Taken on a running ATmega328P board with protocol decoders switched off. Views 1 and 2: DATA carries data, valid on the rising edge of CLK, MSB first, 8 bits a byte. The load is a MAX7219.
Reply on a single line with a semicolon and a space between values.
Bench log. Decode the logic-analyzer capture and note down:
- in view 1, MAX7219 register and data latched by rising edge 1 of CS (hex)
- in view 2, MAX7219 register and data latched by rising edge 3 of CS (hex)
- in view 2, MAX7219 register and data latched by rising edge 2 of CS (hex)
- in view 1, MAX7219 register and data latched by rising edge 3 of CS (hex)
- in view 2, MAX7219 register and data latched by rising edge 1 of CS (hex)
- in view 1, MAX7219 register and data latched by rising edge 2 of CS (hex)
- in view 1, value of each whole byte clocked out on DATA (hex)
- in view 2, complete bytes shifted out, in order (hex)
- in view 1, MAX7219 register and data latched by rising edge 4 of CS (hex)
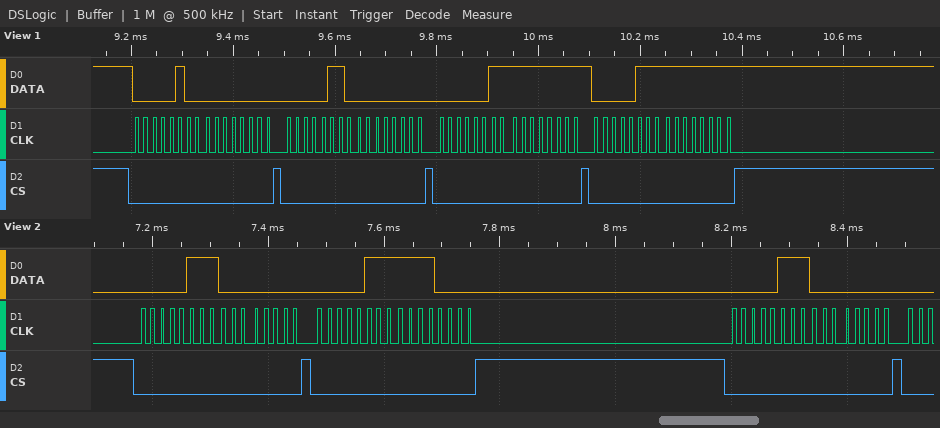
register 0x4, data 0x00; register 0x7, data 0x00; register 0x7, data 0xF0; register 0x3, data 0xFF; register 0x7, data 0x00; register 0x6, data 0x00; 0x04 0x00 0x06 0x00 0x03 0xFF 0x07 0xFF; 07 00 07 F0 07 00; register 0x7, data 0xFF
